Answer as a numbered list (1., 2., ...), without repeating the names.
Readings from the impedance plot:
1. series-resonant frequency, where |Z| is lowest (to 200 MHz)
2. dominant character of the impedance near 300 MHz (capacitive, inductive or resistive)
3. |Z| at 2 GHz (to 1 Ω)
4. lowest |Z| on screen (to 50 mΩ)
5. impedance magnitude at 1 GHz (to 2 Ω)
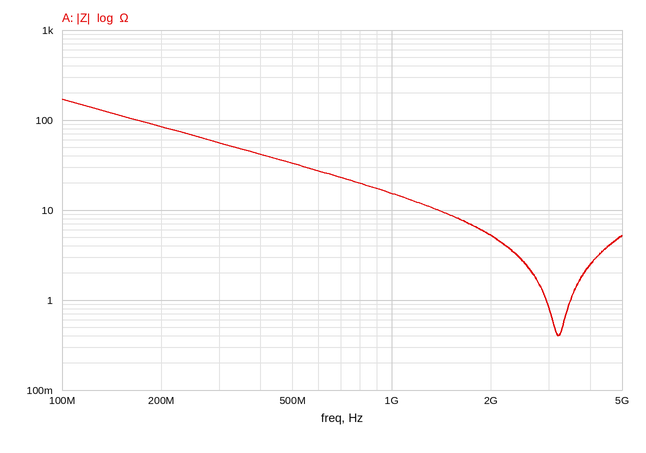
1. 3.2 GHz
2. capacitive
3. 5 Ω
4. 400 mΩ
5. 16 Ω
